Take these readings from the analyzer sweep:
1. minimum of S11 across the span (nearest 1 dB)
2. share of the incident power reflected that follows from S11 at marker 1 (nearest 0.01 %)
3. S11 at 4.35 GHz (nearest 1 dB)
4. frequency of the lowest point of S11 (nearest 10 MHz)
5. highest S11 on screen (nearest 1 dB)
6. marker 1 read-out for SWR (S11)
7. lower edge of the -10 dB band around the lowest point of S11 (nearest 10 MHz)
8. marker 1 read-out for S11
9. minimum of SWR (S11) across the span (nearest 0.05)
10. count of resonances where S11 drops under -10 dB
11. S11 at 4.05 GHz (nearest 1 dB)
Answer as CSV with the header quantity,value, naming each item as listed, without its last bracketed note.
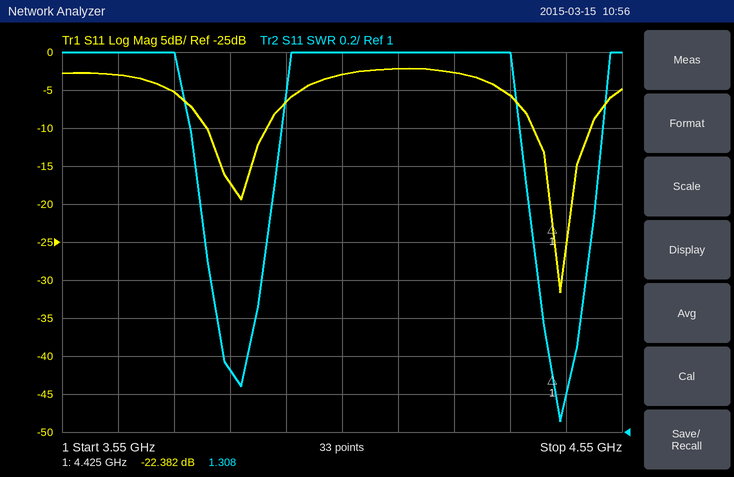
quantity,value
minimum of S11 across the span,-32 dB
share of the incident power reflected that follows from S11 at marker 1,0.58 %
S11 at 4.35 GHz,-6 dB
frequency of the lowest point of S11,4.44 GHz
highest S11 on screen,-2 dB
marker 1 read-out for SWR,1.308
lower edge of the -10 dB band around the lowest point of S11,4.39 GHz
marker 1 read-out for S11,-22.382 dB
minimum of SWR (S11) across the span,1.05
count of resonances where S11 drops under -10 dB,2
S11 at 4.05 GHz,-3 dB
